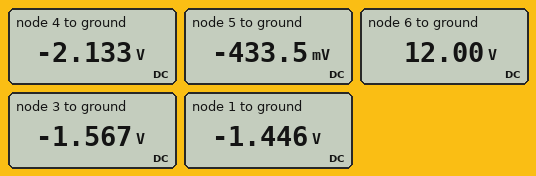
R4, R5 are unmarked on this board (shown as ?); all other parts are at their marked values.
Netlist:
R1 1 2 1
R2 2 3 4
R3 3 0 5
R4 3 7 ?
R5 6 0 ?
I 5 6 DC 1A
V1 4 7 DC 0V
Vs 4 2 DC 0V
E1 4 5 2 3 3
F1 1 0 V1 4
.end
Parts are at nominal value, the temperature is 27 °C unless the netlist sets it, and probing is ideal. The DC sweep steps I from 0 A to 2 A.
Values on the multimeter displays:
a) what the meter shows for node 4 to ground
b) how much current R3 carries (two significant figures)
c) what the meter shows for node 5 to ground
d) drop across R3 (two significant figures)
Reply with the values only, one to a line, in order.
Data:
-2.133 V
310 mA
-433.5 mV
1.6 V
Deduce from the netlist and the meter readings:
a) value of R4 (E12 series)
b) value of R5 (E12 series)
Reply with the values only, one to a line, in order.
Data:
3.3 Ω
12 Ω
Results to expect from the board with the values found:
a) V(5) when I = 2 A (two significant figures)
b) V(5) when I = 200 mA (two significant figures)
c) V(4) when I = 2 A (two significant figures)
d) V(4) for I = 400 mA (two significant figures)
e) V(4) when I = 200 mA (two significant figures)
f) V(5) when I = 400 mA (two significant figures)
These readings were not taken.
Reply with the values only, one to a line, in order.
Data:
-870 mV
-87 mV
-4.3 V
-850 mV
-430 mV
-170 mV
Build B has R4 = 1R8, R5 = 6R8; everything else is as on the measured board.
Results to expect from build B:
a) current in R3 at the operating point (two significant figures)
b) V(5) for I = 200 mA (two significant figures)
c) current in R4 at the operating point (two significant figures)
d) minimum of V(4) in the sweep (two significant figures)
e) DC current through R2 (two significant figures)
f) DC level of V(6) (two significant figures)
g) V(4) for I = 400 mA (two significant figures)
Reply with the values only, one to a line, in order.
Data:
270 mA
-130 mV
180 mA
-3.3 V
83 mA
6.8 V
-660 mV
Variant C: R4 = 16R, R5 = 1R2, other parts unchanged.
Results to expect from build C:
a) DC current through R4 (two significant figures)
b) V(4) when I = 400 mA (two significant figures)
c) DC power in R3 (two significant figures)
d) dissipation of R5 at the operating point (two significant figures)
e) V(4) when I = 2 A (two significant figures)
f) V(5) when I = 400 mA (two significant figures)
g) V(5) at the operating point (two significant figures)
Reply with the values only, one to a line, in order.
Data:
110 mA
-1.8 V
1.5 W
1.2 W
-9.1 V
310 mV
780 mV
